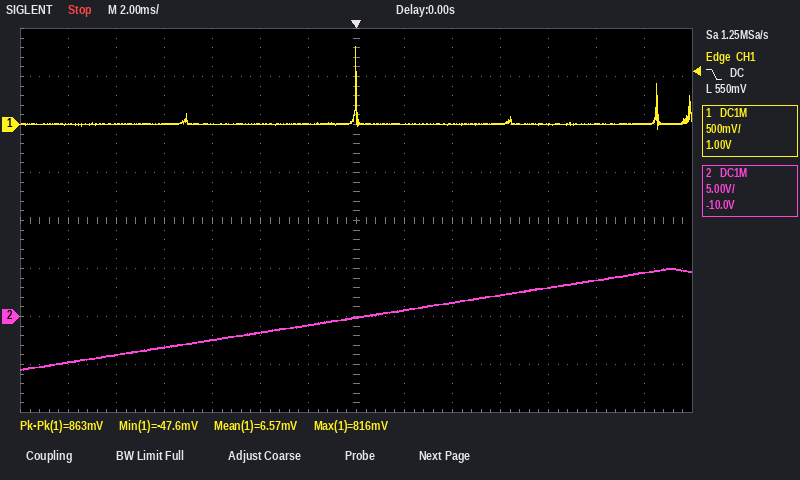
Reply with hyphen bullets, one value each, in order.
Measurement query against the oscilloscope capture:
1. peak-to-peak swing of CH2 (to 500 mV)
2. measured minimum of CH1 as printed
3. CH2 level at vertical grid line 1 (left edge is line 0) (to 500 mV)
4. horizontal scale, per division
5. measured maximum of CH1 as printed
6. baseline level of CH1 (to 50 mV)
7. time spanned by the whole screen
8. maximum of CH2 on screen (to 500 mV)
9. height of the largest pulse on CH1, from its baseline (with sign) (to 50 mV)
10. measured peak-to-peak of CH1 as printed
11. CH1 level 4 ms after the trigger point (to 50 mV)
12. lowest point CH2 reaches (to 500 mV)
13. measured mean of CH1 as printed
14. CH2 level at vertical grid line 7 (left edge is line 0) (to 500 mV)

- 10.5 V
- -47.6 mV
- -5.0 V
- 2 ms
- 816 mV
- 0 mV
- 28 ms
- 5.0 V
- +800 mV
- 863 mV
- 0 mV
- -5.5 V
- 6.57 mV
- 0.0 V
